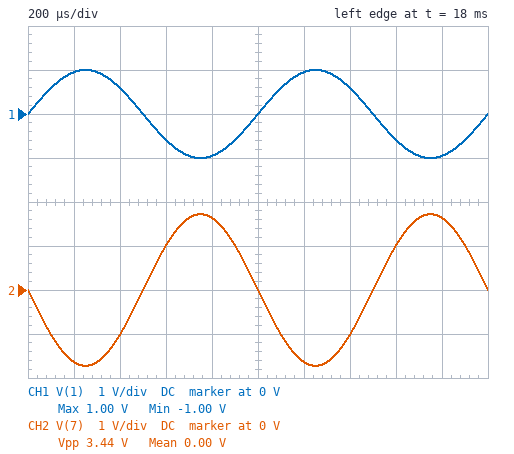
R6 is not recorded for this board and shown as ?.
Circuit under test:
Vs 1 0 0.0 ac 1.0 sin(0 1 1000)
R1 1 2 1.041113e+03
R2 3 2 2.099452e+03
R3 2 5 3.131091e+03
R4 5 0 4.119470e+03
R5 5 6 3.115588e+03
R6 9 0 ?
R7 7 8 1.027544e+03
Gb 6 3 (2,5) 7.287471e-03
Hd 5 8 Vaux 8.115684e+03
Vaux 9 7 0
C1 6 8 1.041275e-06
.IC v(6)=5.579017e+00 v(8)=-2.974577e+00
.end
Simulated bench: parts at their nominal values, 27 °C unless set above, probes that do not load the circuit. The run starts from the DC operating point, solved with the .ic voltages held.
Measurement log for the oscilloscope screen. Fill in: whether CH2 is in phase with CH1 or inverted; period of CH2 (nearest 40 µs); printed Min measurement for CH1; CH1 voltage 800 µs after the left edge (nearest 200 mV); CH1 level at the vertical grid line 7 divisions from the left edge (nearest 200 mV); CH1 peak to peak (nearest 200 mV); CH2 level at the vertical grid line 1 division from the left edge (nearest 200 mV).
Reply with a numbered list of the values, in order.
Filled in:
1. inverted
2. 1.00 ms
3. -1.00 V
4. -1.0 V
5. 600 mV
6. 2.0 V
7. -1.6 V
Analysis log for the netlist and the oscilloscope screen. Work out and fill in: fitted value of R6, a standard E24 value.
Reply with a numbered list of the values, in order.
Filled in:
1. 4.3 kΩ
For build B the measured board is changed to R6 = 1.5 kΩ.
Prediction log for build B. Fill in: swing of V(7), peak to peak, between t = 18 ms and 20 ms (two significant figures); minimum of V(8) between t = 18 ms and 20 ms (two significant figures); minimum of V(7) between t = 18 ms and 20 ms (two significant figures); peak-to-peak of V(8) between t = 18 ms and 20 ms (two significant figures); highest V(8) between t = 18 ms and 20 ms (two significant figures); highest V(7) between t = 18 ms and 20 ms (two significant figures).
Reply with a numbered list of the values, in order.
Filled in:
1. 510 mV
2. -430 mV
3. -250 mV
4. 860 mV
5. 430 mV
6. 250 mV
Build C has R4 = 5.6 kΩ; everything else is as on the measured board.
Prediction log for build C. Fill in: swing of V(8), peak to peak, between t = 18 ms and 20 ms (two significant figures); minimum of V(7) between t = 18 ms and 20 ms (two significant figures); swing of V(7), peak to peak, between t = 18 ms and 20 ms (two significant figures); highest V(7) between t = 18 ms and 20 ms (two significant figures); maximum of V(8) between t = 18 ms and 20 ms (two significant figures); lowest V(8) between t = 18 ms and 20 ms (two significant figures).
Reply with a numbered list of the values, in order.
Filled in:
1. 4.6 V
2. -1.8 V
3. 3.7 V
4. 1.8 V
5. 2.3 V
6. -2.3 V
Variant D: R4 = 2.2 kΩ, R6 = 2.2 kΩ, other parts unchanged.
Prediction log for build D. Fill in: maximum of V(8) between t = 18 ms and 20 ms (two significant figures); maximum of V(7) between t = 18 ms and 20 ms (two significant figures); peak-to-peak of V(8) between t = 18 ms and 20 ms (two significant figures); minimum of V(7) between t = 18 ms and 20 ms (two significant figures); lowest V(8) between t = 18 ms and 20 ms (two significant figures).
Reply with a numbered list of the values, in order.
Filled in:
1. 540 mV
2. 370 mV
3. 1.1 V
4. -370 mV
5. -540 mV
